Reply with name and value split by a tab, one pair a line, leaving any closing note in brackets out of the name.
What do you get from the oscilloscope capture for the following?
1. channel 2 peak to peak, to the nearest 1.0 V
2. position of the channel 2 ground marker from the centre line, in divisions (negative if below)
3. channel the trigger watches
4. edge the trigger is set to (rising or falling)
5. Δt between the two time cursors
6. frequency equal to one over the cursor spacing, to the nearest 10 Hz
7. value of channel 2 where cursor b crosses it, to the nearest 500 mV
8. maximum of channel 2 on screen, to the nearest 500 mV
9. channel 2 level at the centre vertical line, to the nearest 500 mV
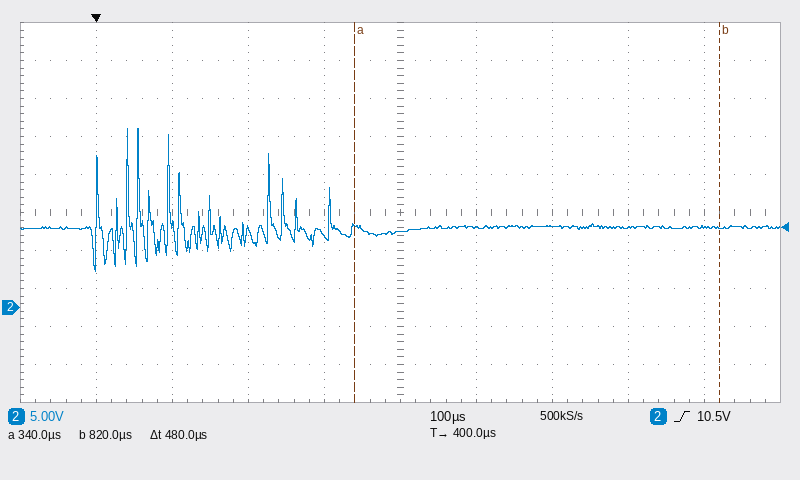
channel 2 peak to peak, to the nearest 1.0 V	19.0 V
position of the channel 2 ground marker from the centre line, in divisions	-2.5 div
channel the trigger watches	channel 2
edge the trigger is set to	rising
Δt between the two time cursors	480 µs
frequency equal to one over the cursor spacing, to the nearest 10 Hz	2.08 kHz
value of channel 2 where cursor b crosses it, to the nearest 500 mV	10.5 V
maximum of channel 2 on screen, to the nearest 500 mV	23.5 V
channel 2 level at the centre vertical line, to the nearest 500 mV	10.0 V
